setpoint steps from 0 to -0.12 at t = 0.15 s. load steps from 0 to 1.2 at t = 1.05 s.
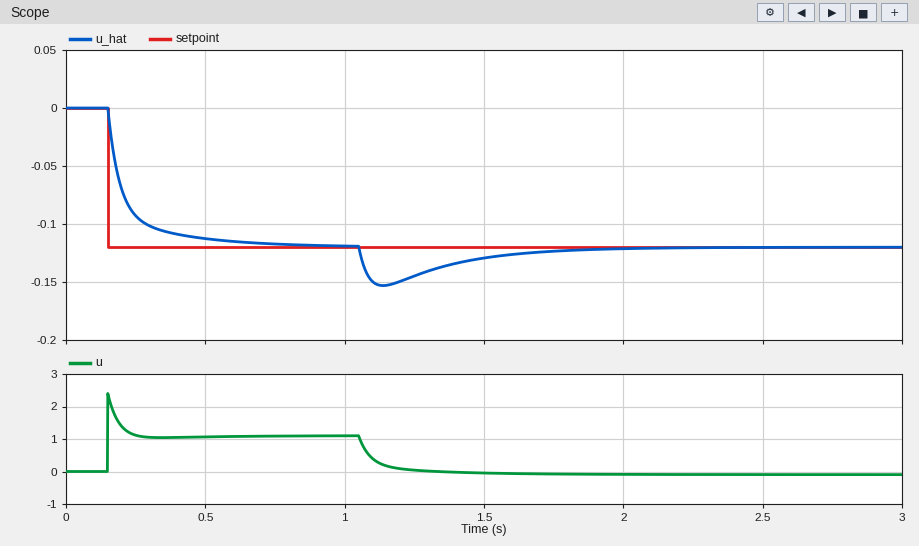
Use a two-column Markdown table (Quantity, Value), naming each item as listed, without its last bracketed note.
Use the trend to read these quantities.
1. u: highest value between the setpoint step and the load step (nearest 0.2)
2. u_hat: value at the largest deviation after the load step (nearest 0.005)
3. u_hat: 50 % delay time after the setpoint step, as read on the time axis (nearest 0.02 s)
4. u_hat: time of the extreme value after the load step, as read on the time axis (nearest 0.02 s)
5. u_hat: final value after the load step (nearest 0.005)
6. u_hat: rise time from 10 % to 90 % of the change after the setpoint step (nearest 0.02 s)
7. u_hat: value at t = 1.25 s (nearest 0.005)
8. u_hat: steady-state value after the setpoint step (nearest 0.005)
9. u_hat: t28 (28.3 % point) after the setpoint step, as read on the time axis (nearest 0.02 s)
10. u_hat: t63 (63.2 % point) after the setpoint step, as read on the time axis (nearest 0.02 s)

| Quantity | Value |
|---|---|
| u: highest value between the setpoint step and the load step | 2.4 |
| u_hat: value at the largest deviation after the load step | -0.155 |
| u_hat: 50 % delay time after the setpoint step, as read on the time axis | 0.18 s |
| u_hat: time of the extreme value after the load step, as read on the time axis | 1.14 s |
| u_hat: final value after the load step | -0.120 |
| u_hat: rise time from 10 % to 90 % of the change after the setpoint step | 0.22 s |
| u_hat: value at t = 1.25 s | -0.145 |
| u_hat: steady-state value after the setpoint step | -0.120 |
| u_hat: t28 (28.3 % point) after the setpoint step, as read on the time axis | 0.16 s |
| u_hat: t63 (63.2 % point) after the setpoint step, as read on the time axis | 0.20 s |
